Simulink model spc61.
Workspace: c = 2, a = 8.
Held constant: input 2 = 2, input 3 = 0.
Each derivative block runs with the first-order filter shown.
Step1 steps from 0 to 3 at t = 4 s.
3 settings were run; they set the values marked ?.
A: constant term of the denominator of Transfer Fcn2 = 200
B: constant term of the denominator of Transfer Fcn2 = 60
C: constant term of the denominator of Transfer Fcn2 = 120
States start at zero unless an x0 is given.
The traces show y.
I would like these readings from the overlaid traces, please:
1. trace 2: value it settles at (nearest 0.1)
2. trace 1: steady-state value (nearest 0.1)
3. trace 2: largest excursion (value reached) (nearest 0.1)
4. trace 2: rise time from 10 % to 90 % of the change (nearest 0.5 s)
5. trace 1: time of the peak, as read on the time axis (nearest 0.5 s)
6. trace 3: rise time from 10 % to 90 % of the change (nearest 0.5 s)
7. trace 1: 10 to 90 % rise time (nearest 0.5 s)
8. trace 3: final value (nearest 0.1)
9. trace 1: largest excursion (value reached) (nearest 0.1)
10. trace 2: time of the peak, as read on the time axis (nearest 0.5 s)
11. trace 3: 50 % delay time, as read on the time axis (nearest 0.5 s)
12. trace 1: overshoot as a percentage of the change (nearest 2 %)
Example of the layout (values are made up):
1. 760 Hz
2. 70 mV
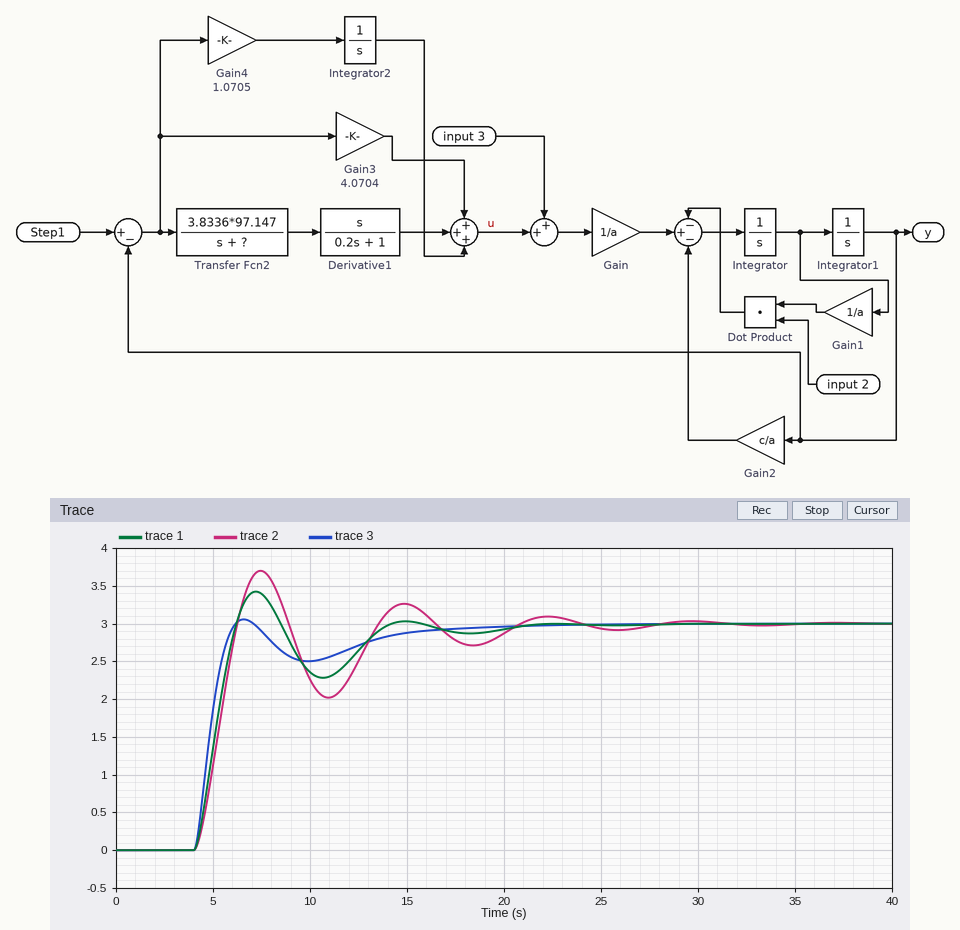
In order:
1. 3.0
2. 3.0
3. 3.7
4. 1.5 s
5. 7.0 s
6. 1.5 s
7. 1.5 s
8. 3.0
9. 3.4
10. 7.5 s
11. 5.0 s
12. 14 %
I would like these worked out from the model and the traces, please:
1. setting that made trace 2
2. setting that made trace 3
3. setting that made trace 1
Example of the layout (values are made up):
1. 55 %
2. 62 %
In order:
1. A
2. B
3. C
